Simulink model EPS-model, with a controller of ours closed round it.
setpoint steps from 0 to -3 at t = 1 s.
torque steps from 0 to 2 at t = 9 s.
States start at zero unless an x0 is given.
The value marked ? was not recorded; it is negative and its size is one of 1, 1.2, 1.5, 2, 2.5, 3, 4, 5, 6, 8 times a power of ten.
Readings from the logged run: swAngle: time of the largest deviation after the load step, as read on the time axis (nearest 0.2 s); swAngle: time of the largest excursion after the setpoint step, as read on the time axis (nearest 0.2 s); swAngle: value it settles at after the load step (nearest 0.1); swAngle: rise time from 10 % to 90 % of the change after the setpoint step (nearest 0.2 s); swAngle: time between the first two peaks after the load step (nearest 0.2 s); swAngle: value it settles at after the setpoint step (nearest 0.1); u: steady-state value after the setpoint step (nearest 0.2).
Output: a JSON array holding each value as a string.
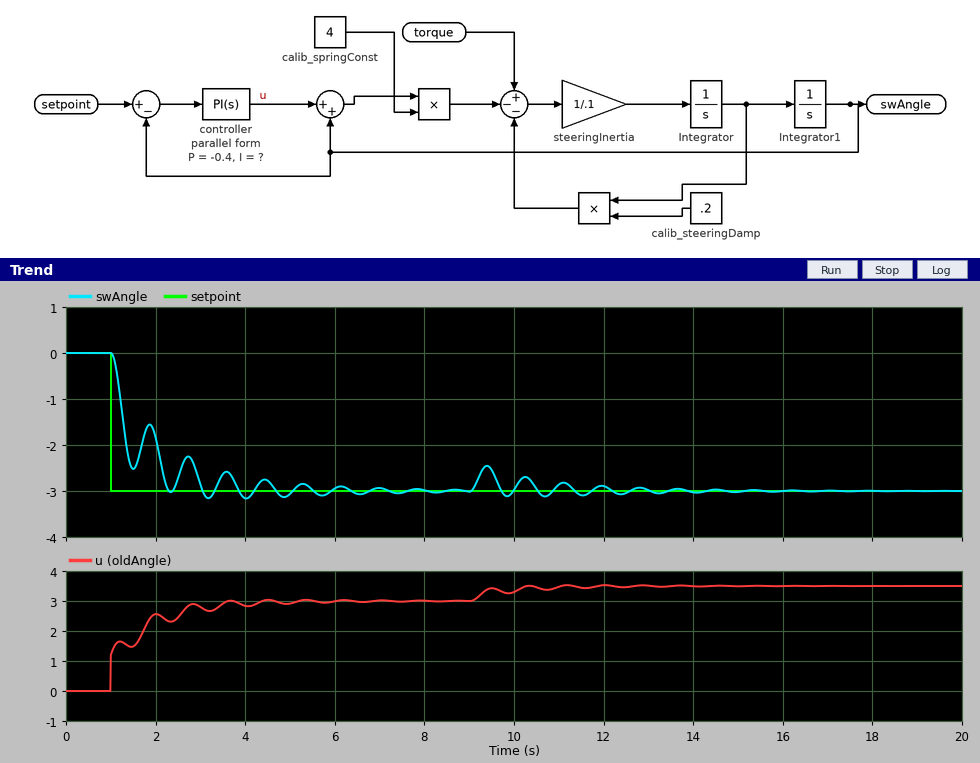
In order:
["9.4 s", "4.0 s", "-3.0", "1.0 s", "0.8 s", "-3.0", "3.0"]
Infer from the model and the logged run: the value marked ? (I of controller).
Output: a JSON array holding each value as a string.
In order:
["-1.5"]
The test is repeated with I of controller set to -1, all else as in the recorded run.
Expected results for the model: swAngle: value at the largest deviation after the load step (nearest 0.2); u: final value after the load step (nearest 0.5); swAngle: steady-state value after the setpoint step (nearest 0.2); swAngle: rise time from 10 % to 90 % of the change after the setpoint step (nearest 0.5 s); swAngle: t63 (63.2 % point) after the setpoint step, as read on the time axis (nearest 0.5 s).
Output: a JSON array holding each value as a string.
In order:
["-2.4", "3.5", "-3.0", "2.0 s", "1.5 s"]
